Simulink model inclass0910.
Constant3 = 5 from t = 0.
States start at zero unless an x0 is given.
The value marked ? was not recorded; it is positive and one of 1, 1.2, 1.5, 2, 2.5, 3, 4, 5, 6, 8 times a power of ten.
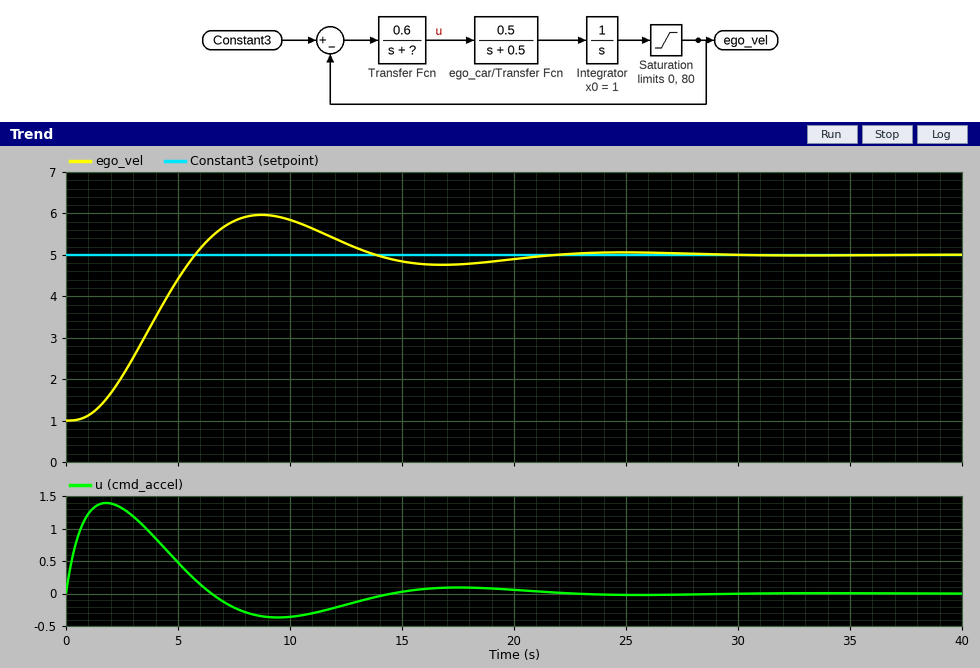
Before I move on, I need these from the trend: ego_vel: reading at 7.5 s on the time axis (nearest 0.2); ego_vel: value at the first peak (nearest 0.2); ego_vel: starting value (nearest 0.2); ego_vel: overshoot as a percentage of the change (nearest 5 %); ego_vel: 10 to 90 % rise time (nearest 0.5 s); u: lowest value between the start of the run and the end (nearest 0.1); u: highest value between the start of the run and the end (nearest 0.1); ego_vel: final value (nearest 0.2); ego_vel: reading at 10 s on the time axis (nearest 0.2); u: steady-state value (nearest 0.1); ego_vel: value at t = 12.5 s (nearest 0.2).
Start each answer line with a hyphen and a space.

- 5.8
- 6.0
- 1.0
- 25 %
- 3.5 s
- -0.4
- 1.4
- 5.0
- 5.8
- 0.0
- 5.2
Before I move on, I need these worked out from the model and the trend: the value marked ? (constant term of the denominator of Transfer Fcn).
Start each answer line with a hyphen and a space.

- 1.5
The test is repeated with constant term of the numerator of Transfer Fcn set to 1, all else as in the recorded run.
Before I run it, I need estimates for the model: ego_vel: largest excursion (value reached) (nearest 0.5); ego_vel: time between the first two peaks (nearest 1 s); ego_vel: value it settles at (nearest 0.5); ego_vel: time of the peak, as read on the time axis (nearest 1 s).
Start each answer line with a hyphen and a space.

- 6.5
- 12 s
- 5.0
- 7 s
